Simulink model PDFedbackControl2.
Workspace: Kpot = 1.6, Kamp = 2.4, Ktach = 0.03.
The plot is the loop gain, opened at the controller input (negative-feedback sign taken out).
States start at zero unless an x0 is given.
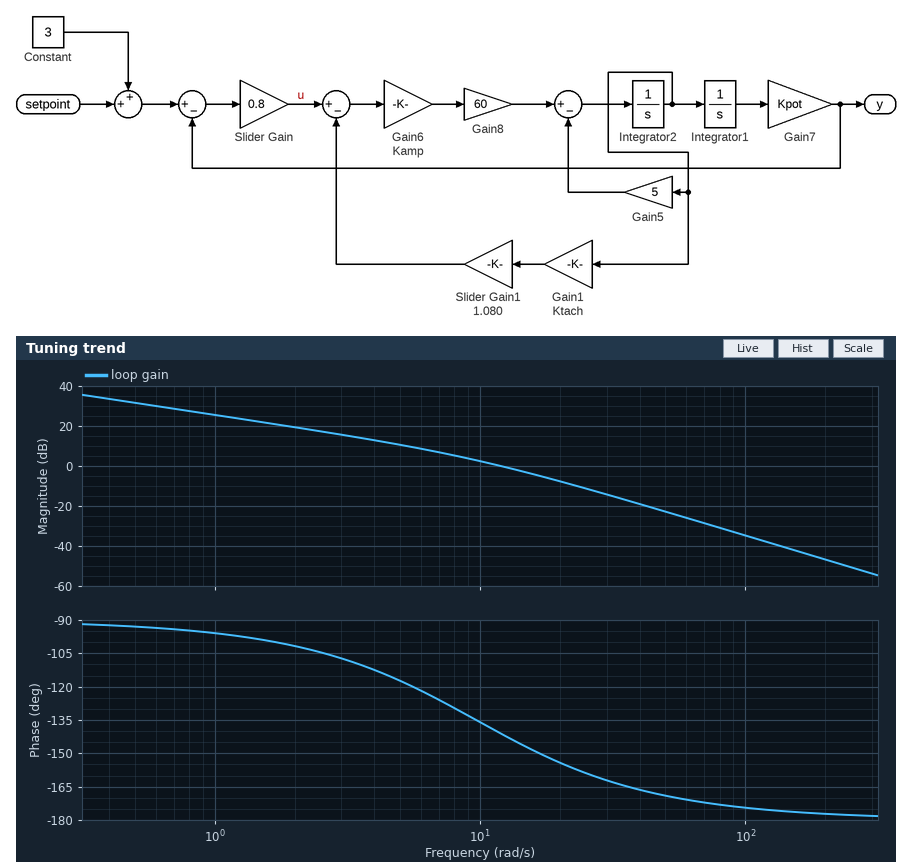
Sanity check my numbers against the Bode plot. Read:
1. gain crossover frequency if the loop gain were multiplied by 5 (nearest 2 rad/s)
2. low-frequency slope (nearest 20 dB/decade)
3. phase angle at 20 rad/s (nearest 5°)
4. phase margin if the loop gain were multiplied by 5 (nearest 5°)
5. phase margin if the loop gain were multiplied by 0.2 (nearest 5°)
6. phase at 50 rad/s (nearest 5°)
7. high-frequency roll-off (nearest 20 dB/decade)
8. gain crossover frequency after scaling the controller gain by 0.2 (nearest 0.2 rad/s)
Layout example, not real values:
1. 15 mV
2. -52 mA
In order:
1. 30 rad/s
2. -20 dB/decade
3. -155°
4. 20°
5. 70°
6. -170°
7. -40 dB/decade
8. 3.6 rad/s
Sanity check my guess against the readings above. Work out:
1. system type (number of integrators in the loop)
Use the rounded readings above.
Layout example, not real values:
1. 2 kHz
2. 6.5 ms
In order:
1. 1
